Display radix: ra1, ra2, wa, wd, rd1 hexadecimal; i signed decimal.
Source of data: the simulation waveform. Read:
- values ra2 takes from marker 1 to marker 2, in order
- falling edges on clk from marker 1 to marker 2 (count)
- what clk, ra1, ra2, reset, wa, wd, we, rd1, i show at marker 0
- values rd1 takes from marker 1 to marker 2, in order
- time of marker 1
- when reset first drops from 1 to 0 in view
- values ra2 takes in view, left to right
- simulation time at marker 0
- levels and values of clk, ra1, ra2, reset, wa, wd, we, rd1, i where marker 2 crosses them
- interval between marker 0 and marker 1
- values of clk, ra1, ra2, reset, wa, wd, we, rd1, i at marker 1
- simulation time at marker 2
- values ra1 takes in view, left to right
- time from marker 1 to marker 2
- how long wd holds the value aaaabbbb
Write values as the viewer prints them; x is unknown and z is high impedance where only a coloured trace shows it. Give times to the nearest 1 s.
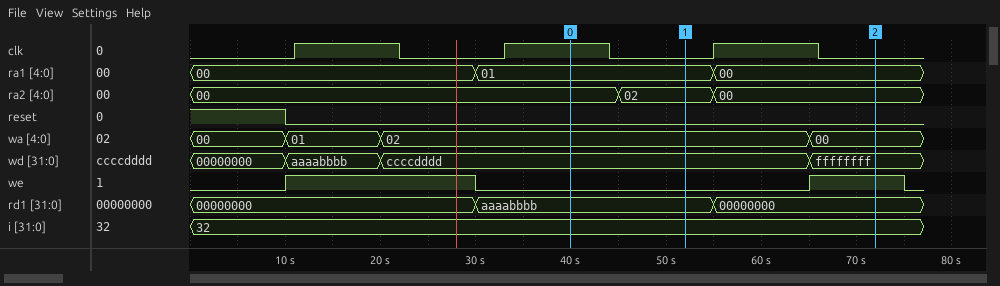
02, 00
1
clk=1, ra1=01, ra2=00, reset=0, wa=02, wd=ccccdddd, we=0, rd1=aaaabbbb, i=32
aaaabbbb, 00000000
52 s
10 s
00, 02, 00
40 s
clk=0, ra1=00, ra2=00, reset=0, wa=00, wd=ffffffff, we=1, rd1=00000000, i=32
12 s
clk=0, ra1=01, ra2=02, reset=0, wa=02, wd=ccccdddd, we=0, rd1=aaaabbbb, i=32
72 s
00, 01, 00
20 s
10 s
